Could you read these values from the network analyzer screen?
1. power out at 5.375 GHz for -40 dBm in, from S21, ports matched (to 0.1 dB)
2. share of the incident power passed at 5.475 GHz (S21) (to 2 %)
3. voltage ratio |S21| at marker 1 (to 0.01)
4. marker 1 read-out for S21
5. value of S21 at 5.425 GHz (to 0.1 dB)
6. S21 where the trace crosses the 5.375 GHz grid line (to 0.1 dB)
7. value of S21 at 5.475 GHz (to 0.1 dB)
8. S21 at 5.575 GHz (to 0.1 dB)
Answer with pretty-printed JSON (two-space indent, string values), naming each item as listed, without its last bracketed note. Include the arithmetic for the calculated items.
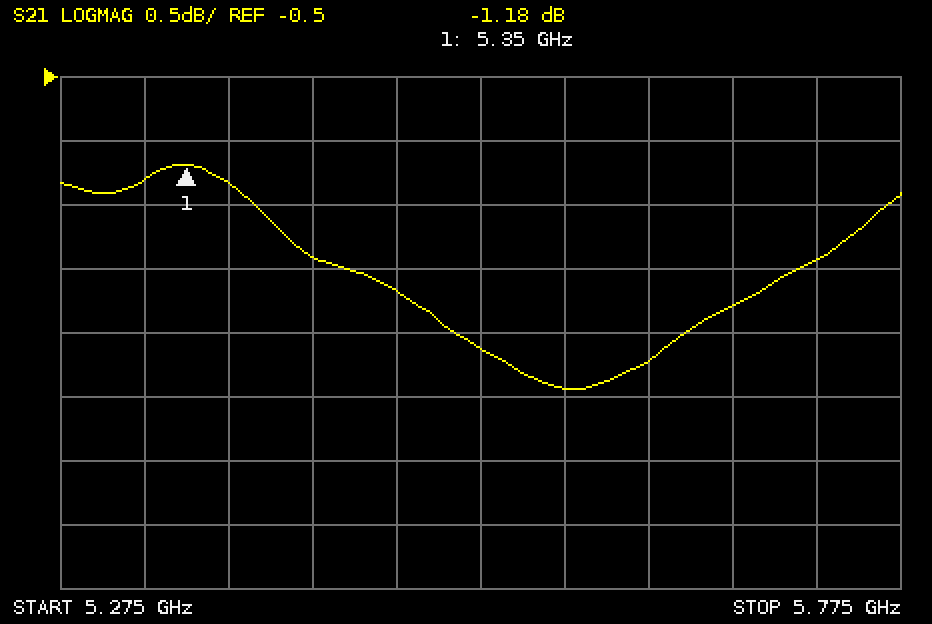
{
  "power out at 5.375 GHz for -40 dBm in, from S21, ports matched": "-40 dBm + (-1.3 dB) = -41.3 dBm",
  "share of the incident power passed at 5.475 GHz (S21)": "10^(-2.2/10) ≈ 60 %",
  "voltage ratio |S21| at marker 1": "10^(-1.18/20) ≈ 0.87",
  "marker 1 read-out for S21": "-1.18 dB",
  "value of S21 at 5.425 GHz": "-1.9 dB",
  "S21 where the trace crosses the 5.375 GHz grid line": "-1.3 dB",
  "value of S21 at 5.475 GHz": "-2.2 dB",
  "S21 at 5.575 GHz": "-2.9 dB"
}
